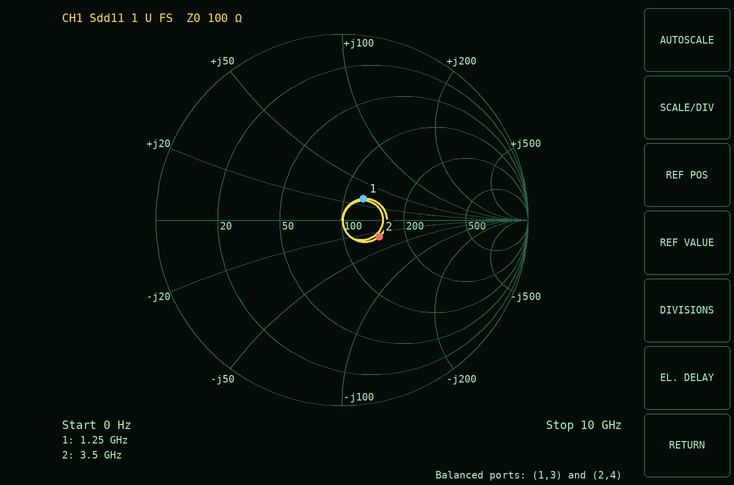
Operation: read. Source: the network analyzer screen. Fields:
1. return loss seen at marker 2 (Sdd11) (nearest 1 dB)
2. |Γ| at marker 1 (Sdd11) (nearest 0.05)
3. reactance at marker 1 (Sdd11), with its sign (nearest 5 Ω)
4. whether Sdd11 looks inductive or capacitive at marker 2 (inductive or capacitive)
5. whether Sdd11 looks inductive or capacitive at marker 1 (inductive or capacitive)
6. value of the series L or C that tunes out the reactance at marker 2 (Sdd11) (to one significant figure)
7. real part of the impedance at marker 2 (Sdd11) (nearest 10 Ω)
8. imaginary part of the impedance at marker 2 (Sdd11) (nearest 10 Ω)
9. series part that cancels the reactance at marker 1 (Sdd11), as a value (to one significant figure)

13 dB
0.15
+30 Ω
capacitive
inductive
1 nH
150 Ω
-30 Ω
4 pF
